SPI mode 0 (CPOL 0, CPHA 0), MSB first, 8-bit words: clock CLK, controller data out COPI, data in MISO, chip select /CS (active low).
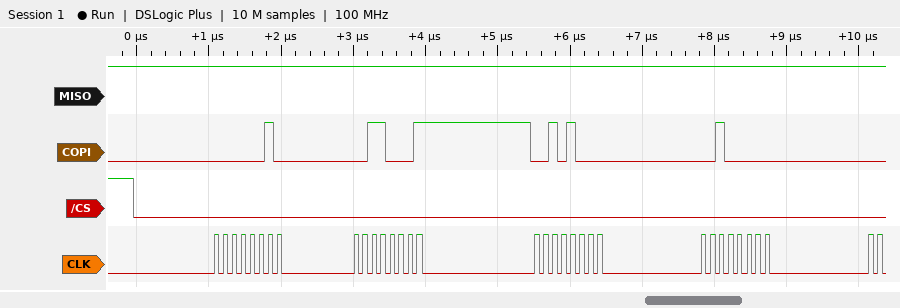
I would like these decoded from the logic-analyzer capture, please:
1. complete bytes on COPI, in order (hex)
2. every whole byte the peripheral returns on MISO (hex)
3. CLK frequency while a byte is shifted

02 31 28 20
FF FF FF FF
8 MHz
